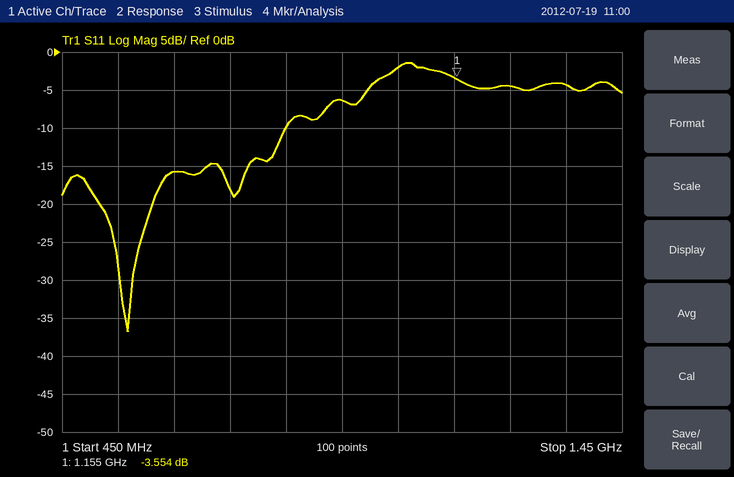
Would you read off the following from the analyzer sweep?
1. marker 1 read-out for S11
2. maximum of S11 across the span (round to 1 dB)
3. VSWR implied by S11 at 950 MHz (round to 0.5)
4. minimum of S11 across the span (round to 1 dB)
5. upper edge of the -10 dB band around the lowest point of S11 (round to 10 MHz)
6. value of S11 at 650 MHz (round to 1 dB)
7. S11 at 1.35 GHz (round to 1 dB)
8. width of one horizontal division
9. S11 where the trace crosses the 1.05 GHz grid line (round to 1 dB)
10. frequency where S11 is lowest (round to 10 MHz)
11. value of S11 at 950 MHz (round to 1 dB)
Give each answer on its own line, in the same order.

-3.554 dB
-1 dB
3.0
-37 dB
850 MHz
-16 dB
-4 dB
100 MHz
-2 dB
570 MHz
-6 dB
